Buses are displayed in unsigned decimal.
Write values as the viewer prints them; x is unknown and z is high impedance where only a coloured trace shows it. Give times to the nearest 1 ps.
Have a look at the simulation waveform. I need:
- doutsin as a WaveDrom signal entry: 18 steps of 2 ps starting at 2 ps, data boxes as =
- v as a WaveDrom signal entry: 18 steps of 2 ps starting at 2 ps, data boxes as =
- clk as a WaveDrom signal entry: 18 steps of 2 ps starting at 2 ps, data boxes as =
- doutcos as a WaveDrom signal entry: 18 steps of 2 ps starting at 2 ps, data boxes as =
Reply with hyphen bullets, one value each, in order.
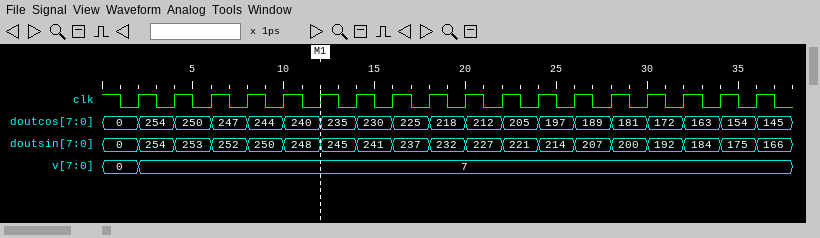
- {name: 'doutsin', wave: '==================', data: '254 253 252 250 248 245 241 237 232 227 221 214 207 200 192 184 175 166'}
- {name: 'v', wave: '=.................', data: '7'}
- {name: 'clk', wave: 'p.................'}
- {name: 'doutcos', wave: '==================', data: '254 250 247 244 240 235 230 225 218 212 205 197 189 181 172 163 154 145'}
